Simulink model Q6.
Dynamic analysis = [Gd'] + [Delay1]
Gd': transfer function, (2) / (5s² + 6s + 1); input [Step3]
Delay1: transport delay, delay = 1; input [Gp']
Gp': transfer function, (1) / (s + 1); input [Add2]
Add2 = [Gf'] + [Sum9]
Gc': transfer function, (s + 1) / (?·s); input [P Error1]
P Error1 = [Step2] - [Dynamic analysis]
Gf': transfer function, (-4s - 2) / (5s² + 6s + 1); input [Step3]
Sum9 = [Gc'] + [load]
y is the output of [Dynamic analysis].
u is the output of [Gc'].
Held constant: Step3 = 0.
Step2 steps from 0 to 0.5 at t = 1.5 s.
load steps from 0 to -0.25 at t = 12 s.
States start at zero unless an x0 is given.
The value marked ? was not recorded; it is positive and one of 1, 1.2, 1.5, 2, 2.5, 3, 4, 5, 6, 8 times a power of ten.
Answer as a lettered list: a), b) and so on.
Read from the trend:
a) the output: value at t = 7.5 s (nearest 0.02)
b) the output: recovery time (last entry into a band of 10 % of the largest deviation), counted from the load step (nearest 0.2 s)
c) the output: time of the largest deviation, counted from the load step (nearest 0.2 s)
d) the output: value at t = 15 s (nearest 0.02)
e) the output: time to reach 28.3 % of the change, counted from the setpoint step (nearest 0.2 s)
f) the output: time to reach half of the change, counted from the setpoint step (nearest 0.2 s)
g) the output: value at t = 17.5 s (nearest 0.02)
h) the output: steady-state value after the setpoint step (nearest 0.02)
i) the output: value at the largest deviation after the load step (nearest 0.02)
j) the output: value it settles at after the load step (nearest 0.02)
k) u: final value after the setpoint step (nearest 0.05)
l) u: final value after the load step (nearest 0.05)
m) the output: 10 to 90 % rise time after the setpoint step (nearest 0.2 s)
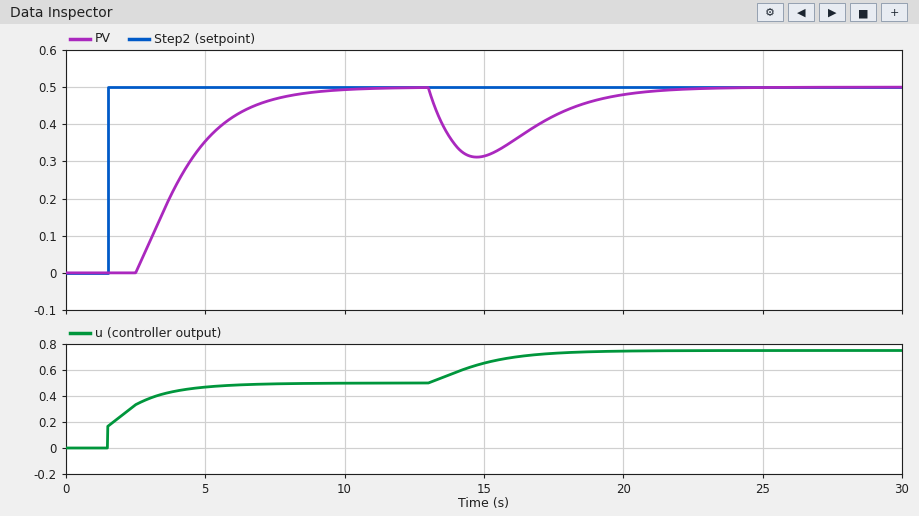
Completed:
a) 0.46
b) 8.2 s
c) 2.8 s
d) 0.32
e) 1.8 s
f) 2.6 s
g) 0.42
h) 0.50
i) 0.32
j) 0.50
k) 0.50
l) 0.75
m) 4.0 s
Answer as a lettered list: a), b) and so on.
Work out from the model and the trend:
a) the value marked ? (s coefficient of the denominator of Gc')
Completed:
a) 3
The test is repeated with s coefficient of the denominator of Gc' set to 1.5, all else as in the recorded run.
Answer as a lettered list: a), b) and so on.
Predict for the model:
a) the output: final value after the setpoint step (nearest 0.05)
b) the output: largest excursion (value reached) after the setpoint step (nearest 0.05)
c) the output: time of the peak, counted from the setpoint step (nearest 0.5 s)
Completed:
a) 0.50
b) 0.60
c) 3.5 s
